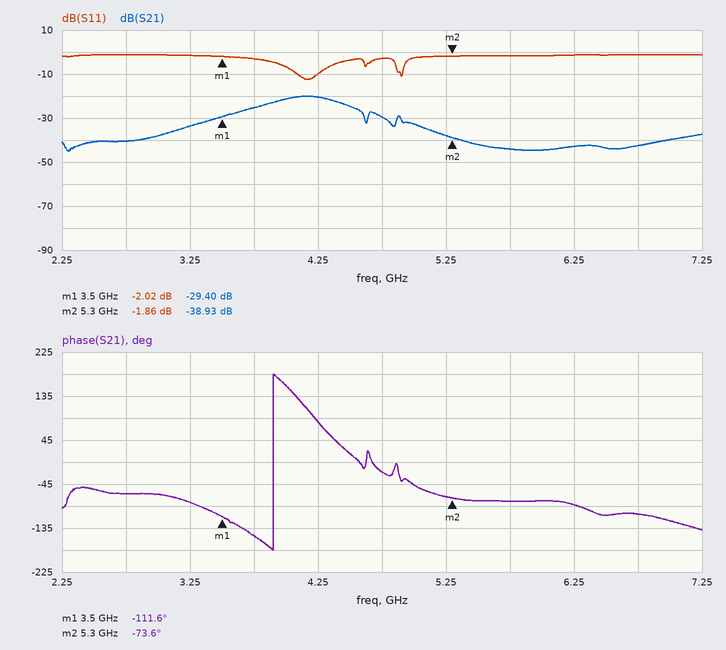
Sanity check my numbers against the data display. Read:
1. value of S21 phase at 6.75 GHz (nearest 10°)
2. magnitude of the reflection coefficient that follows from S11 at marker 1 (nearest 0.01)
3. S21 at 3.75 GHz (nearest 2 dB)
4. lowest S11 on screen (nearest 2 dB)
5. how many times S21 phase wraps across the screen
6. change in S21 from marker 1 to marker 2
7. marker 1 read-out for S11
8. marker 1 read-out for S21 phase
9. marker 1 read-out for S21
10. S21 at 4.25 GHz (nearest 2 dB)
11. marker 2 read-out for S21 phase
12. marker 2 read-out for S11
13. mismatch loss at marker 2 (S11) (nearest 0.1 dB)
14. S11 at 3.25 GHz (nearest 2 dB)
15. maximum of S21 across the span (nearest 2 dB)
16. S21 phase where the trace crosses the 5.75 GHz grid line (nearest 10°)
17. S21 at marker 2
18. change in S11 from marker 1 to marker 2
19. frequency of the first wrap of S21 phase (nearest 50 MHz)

-110°
0.79
-26 dB
-12 dB
1
-9.53 dB
-2.02 dB
-111.6°
-29.40 dB
-20 dB
-73.6°
-1.86 dB
4.6 dB
-2 dB
-20 dB
-80°
-38.93 dB
0.16 dB
3.90 GHz
